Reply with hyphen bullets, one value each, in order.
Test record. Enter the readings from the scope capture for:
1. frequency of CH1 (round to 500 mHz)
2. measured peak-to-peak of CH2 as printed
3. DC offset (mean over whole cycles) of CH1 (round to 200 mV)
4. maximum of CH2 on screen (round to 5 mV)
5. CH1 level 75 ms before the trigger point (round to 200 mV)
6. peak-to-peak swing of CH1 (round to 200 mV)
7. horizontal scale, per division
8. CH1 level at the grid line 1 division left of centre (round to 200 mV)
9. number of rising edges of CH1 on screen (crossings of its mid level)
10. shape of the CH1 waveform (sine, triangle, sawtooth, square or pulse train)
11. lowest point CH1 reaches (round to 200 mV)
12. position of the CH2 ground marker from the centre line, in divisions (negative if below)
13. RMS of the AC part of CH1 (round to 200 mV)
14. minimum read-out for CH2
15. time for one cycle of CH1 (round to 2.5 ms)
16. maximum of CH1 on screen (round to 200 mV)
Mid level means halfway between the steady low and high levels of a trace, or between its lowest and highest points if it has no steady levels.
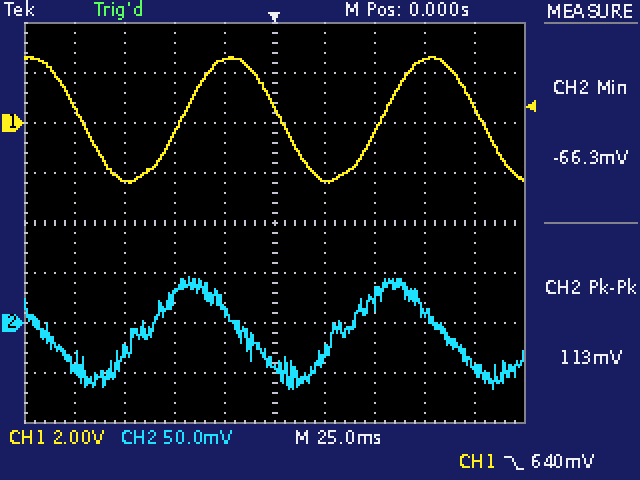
- 10.0 Hz
- 113 mV
- 200 mV
- 45 mV
- -2.2 V
- 5.0 V
- 25 ms
- 2.6 V
- 2
- sine
- -2.4 V
- -2.0 div
- 1.8 V
- -66.3 mV
- 100.0 ms
- 2.6 V
